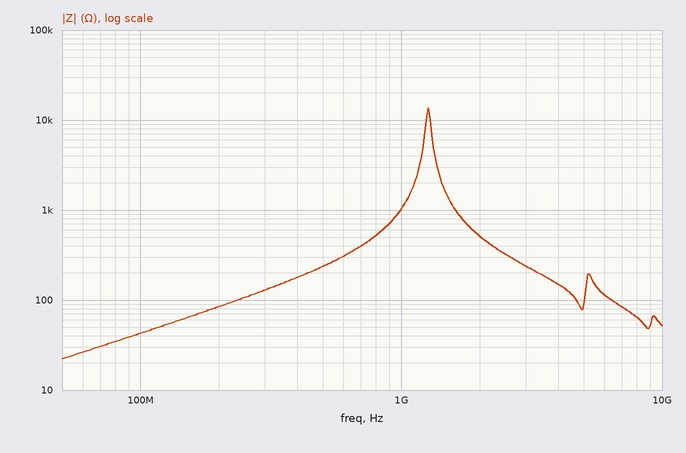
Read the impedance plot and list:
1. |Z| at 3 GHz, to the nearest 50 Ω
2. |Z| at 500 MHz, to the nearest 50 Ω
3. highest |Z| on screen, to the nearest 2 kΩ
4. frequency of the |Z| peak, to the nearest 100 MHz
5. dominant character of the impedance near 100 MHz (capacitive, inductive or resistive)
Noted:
250 Ω
250 Ω
14 kΩ
1.3 GHz
inductive
